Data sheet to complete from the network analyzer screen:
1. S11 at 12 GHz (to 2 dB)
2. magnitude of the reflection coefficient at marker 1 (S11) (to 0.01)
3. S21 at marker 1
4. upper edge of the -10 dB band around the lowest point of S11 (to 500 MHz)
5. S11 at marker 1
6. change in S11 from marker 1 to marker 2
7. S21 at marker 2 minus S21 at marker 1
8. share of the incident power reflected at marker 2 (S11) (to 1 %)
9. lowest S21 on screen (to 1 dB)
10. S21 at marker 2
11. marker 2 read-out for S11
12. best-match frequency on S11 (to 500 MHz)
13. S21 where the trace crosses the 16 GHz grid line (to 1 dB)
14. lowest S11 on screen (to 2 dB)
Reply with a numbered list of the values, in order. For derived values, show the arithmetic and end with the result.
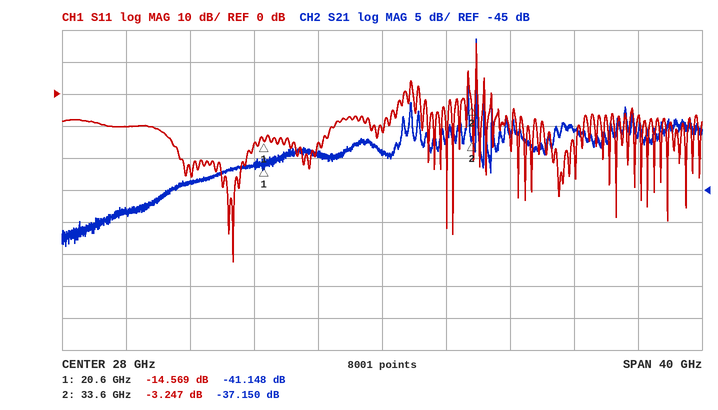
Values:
1. -10 dB
2. 10^(-14.569/20) ≈ 0.19
3. -41.148 dB
4. 25.0 GHz
5. -14.569 dB
6. -3.247 − (-14.569) = 11.322 dB
7. -37.15 − (-41.148) = 3.998 dB
8. 10^(-3.247/10) ≈ 47 %
9. -54 dB
10. -37.150 dB
11. -3.247 dB
12. 18.5 GHz
13. -44 dB
14. -52 dB
